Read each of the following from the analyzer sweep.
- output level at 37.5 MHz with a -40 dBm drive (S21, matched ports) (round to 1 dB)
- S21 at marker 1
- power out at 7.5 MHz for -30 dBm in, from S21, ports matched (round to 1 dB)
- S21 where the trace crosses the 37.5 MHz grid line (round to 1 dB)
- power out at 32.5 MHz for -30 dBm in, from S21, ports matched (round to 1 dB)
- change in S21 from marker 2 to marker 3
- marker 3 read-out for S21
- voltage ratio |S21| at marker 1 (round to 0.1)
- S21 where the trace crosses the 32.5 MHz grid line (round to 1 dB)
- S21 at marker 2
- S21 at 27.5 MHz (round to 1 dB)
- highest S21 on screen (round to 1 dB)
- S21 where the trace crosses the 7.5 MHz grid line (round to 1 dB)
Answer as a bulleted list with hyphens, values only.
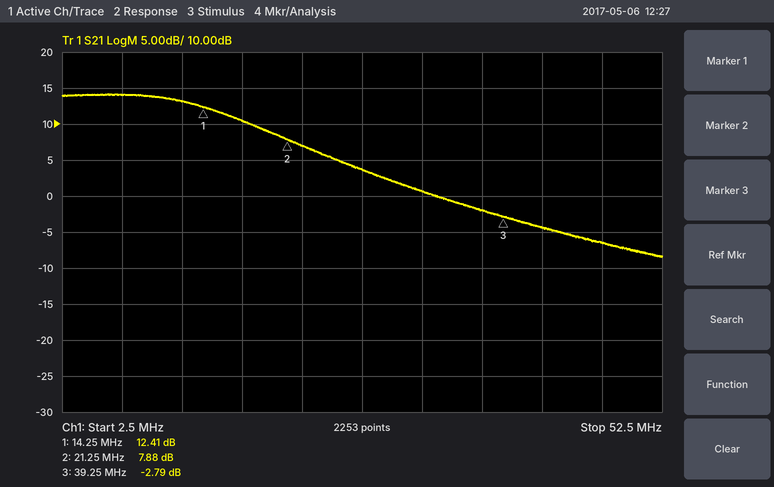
- -42 dBm
- 12.41 dB
- -16 dBm
- -2 dB
- -29 dBm
- -10.67 dB
- -2.79 dB
- 4.2
- 1 dB
- 7.88 dB
- 4 dB
- 14 dB
- 14 dB
